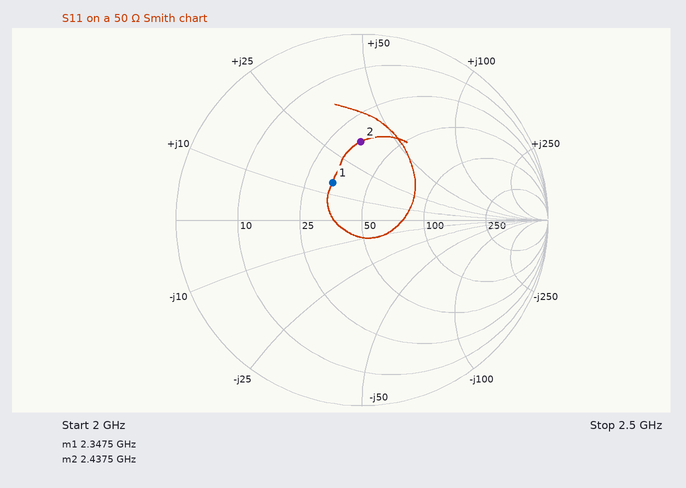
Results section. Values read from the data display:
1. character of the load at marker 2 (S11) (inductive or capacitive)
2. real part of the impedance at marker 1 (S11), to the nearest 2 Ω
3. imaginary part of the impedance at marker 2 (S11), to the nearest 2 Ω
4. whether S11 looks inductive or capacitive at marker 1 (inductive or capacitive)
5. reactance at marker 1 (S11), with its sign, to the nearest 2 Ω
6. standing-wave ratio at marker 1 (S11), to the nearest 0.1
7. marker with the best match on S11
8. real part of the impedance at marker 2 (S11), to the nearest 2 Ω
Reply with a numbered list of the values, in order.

1. inductive
2. 34 Ω
3. +36 Ω
4. inductive
5. +14 Ω
6. 1.7
7. marker 1
8. 34 Ω
